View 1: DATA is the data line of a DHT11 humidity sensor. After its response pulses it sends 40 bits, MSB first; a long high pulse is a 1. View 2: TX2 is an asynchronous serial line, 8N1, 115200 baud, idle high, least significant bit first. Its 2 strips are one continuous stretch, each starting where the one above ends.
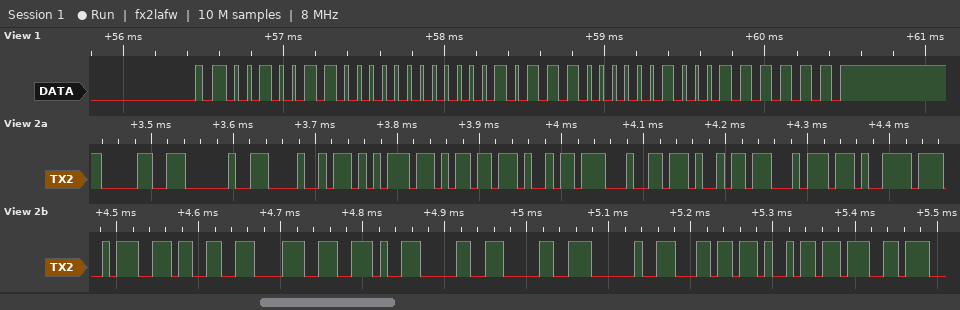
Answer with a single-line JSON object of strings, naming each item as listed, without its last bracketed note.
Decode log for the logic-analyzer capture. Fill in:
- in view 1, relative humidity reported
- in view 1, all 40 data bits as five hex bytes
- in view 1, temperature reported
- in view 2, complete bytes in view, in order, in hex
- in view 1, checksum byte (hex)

{"in view 1, relative humidity reported": "38 %", "in view 1, all 40 data bits as five hex bytes": "26 00 17 02 3F", "in view 1, temperature reported": "23.2 °C", "in view 2, complete bytes in view, in order, in hex": "30 20 48 75 6D 69 64 69 74 79 3A 33 38 2E 30 30 20 6C 69 67", "in view 1, checksum byte": "0x3F"}
